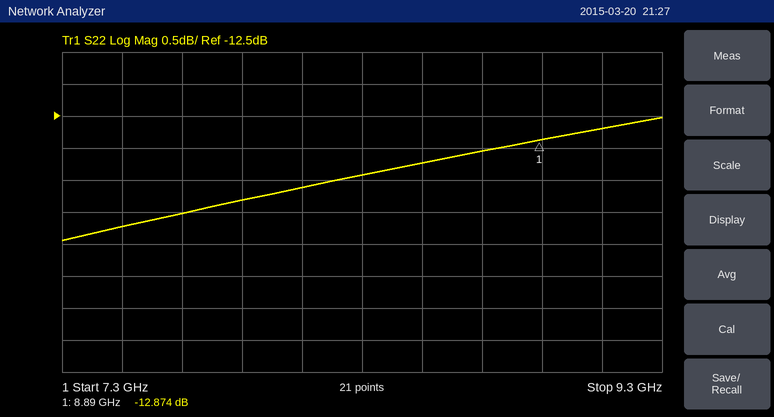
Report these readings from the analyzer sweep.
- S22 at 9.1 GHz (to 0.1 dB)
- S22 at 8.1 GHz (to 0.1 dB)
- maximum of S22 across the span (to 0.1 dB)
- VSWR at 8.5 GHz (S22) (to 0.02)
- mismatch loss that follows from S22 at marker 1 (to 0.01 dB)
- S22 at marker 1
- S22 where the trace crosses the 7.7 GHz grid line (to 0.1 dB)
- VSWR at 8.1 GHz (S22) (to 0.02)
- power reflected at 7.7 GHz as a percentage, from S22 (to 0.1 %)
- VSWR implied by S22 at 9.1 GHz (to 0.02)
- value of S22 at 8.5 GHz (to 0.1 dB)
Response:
-12.7 dB
-13.6 dB
-12.5 dB
1.56
0.23 dB
-12.874 dB
-14.0 dB
1.52
4.0 %
1.60
-13.2 dB
